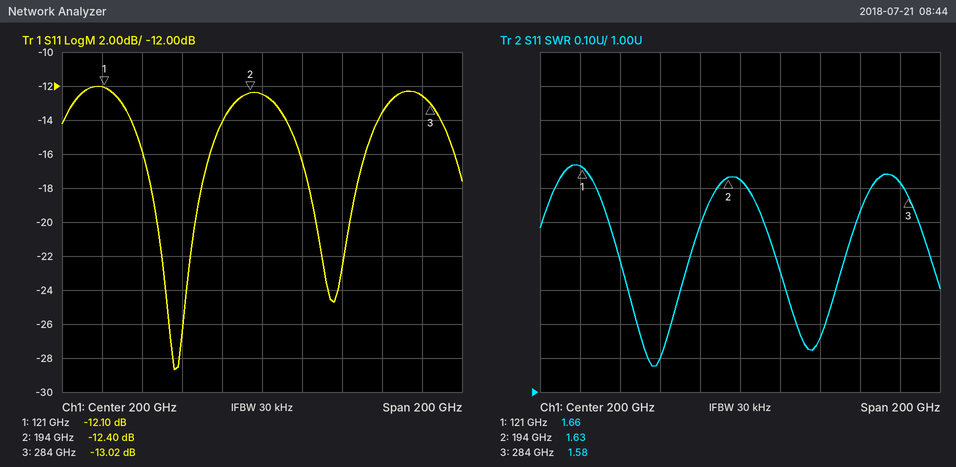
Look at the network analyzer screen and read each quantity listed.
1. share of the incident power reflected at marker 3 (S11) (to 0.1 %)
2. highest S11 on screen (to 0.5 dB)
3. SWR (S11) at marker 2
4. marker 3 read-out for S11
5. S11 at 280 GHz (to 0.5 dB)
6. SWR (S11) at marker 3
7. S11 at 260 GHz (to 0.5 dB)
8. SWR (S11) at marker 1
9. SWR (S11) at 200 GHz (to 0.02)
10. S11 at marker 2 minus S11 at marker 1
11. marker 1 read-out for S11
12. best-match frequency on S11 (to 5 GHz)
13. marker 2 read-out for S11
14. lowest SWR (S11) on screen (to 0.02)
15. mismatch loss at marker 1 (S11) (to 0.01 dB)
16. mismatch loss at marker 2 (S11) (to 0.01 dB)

5.0 %
-12.0 dB
1.63
-13.02 dB
-12.5 dB
1.58
-13.5 dB
1.66
1.62
-0.30 dB
-12.10 dB
155 GHz
-12.40 dB
1.08
0.28 dB
0.26 dB
